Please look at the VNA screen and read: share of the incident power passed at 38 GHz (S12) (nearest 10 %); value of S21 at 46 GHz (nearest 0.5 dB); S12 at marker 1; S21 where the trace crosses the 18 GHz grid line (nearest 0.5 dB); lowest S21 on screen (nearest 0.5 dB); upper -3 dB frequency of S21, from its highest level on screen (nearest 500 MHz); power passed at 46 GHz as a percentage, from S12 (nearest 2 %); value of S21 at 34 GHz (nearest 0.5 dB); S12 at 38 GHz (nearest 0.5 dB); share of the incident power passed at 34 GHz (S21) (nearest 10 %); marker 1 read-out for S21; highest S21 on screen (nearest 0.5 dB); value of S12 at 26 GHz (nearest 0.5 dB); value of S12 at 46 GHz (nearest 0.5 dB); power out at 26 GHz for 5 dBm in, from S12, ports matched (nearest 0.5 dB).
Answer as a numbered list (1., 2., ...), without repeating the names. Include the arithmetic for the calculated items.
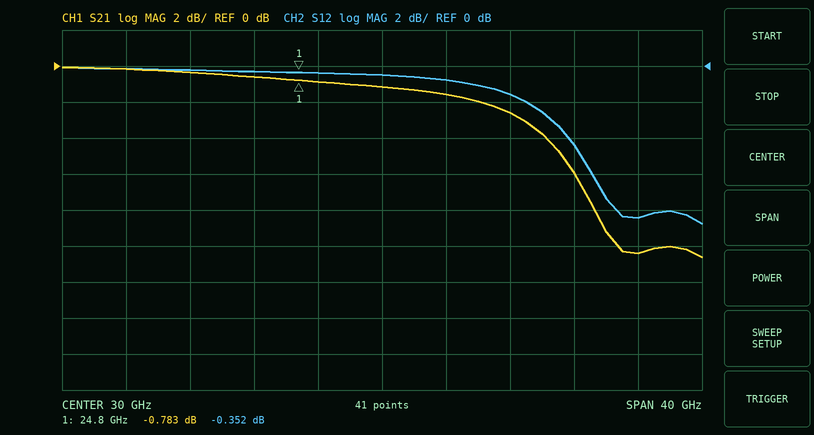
1. 10^(-1.5/10) ≈ 70.8 %, so 70 % to the nearest 10 %
2. -10.5 dB
3. -0.352 dB
4. -0.5 dB
5. -10.5 dB
6. 39.0 GHz
7. 10^(-8.5/10) ≈ 14 %
8. -1.5 dB
9. -1.5 dB
10. 10^(-1.5/10) ≈ 70.8 %, so 70 % to the nearest 10 %
11. -0.783 dB
12. 0.0 dB
13. -0.5 dB
14. -8.5 dB
15. 5 dBm + (-0.5 dB) = 4.5 dBm
